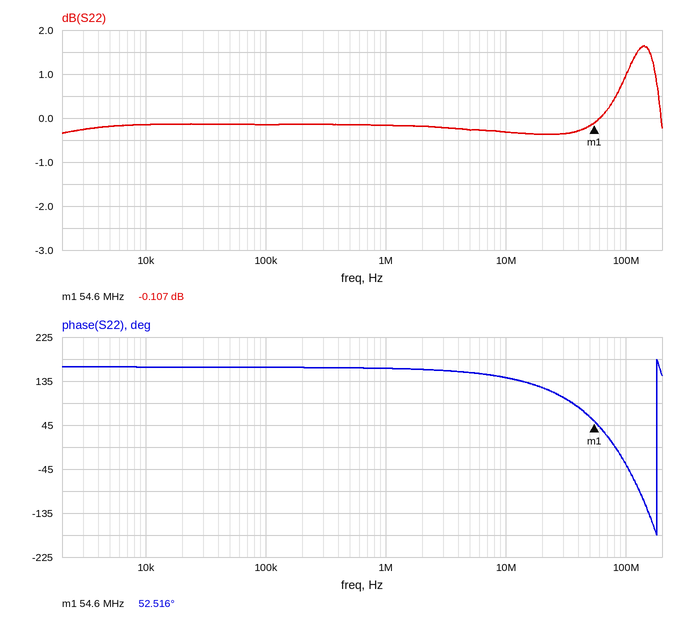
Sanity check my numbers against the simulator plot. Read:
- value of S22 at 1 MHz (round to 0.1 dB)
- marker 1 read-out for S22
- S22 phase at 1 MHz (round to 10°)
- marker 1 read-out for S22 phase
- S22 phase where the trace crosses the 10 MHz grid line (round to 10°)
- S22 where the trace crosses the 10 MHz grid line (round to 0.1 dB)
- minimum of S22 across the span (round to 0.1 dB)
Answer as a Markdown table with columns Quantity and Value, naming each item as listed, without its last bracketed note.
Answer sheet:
| Quantity | Value |
|---|---|
| value of S22 at 1 MHz | -0.2 dB |
| marker 1 read-out for S22 | -0.107 dB |
| S22 phase at 1 MHz | 160° |
| marker 1 read-out for S22 phase | 52.516° |
| S22 phase where the trace crosses the 10 MHz grid line | 140° |
| S22 where the trace crosses the 10 MHz grid line | -0.3 dB |
| minimum of S22 across the span | -0.4 dB |
